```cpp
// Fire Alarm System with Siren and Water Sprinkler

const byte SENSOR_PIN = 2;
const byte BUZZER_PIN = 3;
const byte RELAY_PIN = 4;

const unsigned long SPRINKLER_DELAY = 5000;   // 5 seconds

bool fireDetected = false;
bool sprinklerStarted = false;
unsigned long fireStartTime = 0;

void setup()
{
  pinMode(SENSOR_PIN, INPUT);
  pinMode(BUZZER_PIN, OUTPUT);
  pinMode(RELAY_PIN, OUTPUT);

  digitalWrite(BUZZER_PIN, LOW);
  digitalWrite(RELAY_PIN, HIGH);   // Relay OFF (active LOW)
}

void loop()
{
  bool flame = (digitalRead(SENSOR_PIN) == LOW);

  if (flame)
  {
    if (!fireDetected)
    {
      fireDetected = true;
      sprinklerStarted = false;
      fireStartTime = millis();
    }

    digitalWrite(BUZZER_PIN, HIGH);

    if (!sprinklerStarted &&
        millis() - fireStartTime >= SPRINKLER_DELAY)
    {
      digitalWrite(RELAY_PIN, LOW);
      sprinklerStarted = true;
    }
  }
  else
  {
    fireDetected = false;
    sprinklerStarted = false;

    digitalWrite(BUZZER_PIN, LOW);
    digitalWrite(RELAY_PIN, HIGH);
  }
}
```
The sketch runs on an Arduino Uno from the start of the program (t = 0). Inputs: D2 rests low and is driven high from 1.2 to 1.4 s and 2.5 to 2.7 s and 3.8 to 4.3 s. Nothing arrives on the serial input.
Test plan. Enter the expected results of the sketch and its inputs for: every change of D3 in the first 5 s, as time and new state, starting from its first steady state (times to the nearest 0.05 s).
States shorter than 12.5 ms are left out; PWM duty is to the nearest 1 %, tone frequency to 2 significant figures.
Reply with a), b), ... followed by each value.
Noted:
a) 0 s high; 1.2 s low; 1.4 s high; 2.5 s low; 2.7 s high; 3.8 s low; 4.3 s high
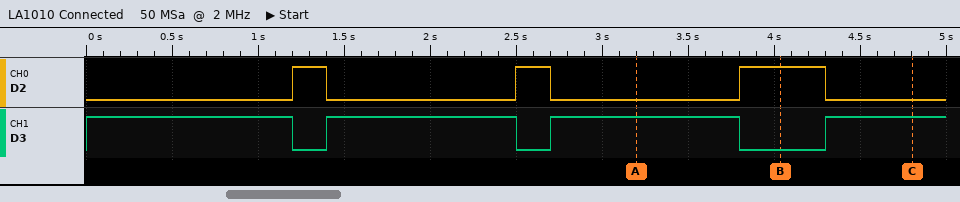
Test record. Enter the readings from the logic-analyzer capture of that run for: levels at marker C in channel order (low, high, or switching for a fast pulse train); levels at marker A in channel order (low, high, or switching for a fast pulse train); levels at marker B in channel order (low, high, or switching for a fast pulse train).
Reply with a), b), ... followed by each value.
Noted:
a) D2 low, D3 high
b) D2 low, D3 high
c) D2 high, D3 low
